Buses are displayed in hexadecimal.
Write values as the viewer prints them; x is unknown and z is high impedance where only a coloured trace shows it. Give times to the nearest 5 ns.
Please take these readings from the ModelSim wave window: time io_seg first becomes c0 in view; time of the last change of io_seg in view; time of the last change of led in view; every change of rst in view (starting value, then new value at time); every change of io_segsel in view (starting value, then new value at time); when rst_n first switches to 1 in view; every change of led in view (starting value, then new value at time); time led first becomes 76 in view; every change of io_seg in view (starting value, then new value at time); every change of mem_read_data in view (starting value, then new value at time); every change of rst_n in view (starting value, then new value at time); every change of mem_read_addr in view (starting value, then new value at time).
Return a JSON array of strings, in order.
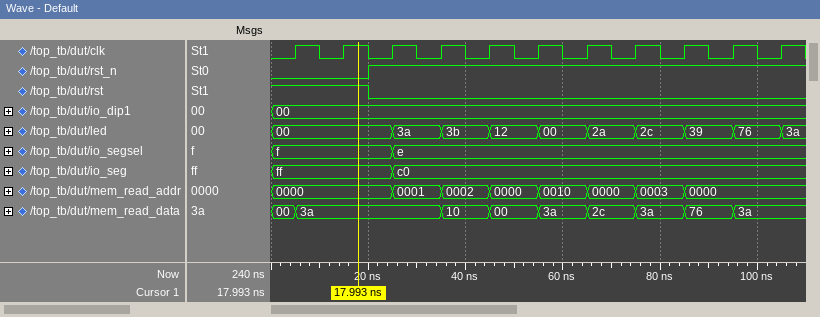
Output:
["25 ns", "25 ns", "105 ns", "1, 0 at 20 ns", "f, e at 25 ns", "20 ns", "00, 3a at 25 ns, 3b at 35 ns, 12 at 45 ns, 00 at 55 ns, 2a at 65 ns, 2c at 75 ns, 39 at 85 ns, 76 at 95 ns, 3a at 105 ns", "95 ns", "ff, c0 at 25 ns", "00, 3a at 5 ns, 10 at 35 ns, 00 at 45 ns, 3a at 55 ns, 2c at 65 ns, 3a at 75 ns, 76 at 85 ns, 3a at 95 ns", "0, 1 at 20 ns", "0000, 0001 at 25 ns, 0002 at 35 ns, 0000 at 45 ns, 0010 at 55 ns, 0000 at 65 ns, 0003 at 75 ns, 0000 at 85 ns"]
